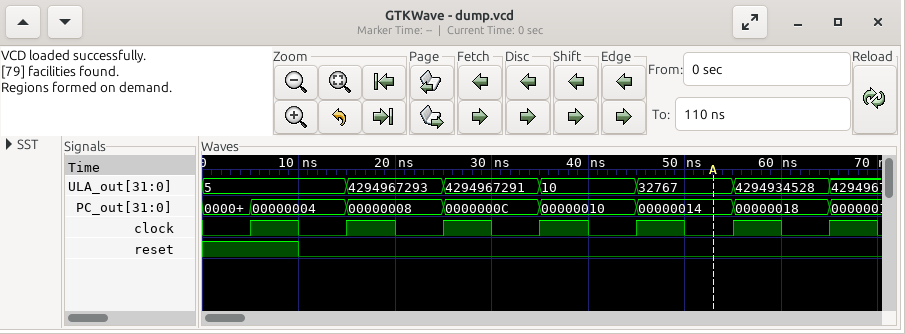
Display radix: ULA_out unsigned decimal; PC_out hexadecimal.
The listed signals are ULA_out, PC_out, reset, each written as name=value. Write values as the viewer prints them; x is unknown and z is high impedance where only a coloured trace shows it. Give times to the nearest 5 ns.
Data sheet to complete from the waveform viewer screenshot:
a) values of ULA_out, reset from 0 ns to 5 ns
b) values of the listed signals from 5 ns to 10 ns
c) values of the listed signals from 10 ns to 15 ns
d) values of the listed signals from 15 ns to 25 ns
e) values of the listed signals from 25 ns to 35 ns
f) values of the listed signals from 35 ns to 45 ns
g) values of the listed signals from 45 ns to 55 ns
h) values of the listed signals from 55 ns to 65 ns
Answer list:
ULA_out=5, reset=1
ULA_out=5, PC_out=00000004, reset=1
ULA_out=5, PC_out=00000004, reset=0
ULA_out=4294967293, PC_out=00000008, reset=0
ULA_out=4294967291, PC_out=0000000C, reset=0
ULA_out=10, PC_out=00000010, reset=0
ULA_out=32767, PC_out=00000014, reset=0
ULA_out=4294934528, PC_out=00000018, reset=0
